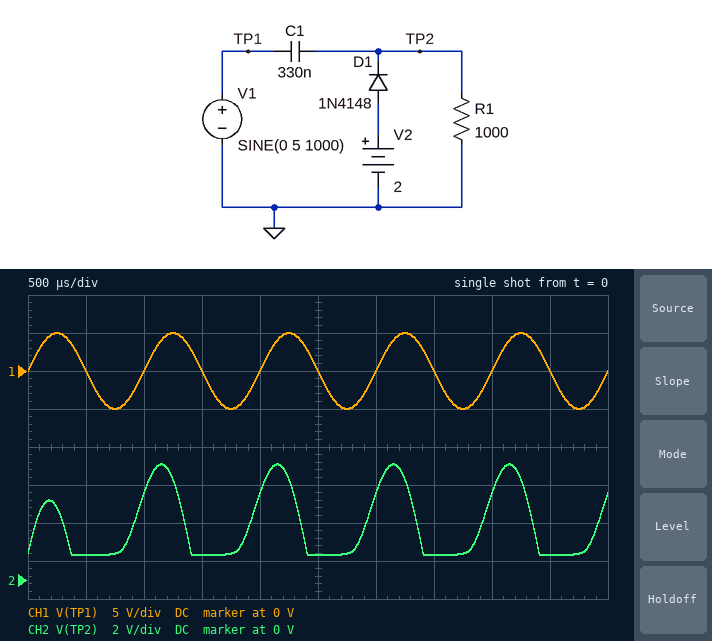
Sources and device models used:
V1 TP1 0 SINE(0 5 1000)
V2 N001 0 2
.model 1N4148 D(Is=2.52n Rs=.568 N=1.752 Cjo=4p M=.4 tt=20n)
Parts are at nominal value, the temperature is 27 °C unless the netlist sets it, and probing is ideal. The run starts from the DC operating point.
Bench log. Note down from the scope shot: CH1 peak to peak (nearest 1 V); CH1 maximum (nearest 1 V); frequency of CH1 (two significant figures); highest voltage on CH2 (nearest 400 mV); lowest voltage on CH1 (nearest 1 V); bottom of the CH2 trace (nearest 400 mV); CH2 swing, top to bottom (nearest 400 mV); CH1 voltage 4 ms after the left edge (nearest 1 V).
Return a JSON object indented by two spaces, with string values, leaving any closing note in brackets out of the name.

{
  "CH1 peak to peak": "10 V",
  "CH1 maximum": "5 V",
  "frequency of CH1": "1.0 kHz",
  "highest voltage on CH2": "6.0 V",
  "lowest voltage on CH1": "-5 V",
  "bottom of the CH2 trace": "1.2 V",
  "CH2 swing, top to bottom": "4.8 V",
  "CH1 voltage 4 ms after the left edge": "0 V"
}
